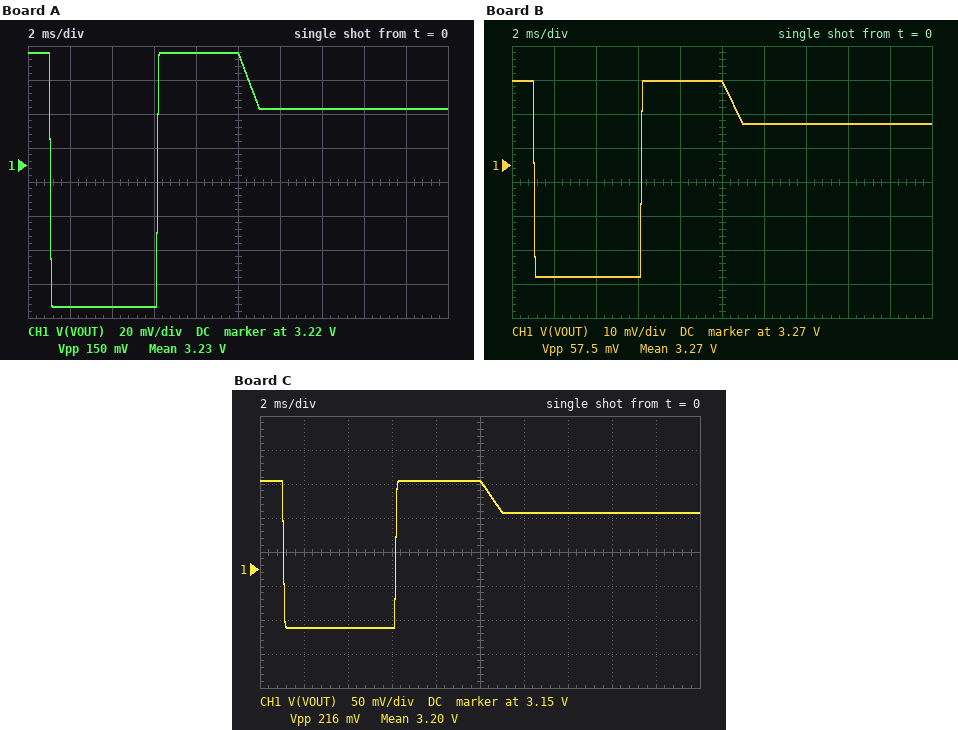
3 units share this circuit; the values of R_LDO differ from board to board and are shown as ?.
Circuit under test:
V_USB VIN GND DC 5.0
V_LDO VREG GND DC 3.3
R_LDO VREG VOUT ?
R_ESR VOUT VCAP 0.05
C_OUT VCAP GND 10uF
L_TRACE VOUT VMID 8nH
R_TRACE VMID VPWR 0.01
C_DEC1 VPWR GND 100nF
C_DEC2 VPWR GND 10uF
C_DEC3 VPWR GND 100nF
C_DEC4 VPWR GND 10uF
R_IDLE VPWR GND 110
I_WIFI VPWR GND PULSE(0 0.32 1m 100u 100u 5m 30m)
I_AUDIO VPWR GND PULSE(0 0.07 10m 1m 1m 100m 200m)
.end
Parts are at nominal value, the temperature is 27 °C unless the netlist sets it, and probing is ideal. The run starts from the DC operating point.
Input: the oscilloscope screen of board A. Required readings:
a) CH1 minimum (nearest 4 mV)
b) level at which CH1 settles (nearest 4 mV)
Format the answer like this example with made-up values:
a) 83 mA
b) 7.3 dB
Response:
a) 3.136 V
b) 3.252 V
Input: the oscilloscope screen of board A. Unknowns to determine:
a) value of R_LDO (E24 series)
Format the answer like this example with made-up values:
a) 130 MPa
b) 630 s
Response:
a) 0.47 Ω
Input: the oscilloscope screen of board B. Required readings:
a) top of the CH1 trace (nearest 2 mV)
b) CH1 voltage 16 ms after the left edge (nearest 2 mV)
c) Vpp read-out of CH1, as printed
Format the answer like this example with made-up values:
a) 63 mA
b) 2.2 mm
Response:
a) 3.294 V
b) 3.282 V
c) 57.5 mV
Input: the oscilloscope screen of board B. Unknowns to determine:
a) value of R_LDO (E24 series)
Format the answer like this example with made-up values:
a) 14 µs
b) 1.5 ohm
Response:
a) 0.18 Ω
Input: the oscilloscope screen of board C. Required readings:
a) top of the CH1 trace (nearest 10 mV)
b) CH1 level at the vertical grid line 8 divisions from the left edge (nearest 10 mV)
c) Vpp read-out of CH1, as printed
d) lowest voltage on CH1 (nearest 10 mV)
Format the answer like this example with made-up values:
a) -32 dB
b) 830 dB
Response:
a) 3.28 V
b) 3.23 V
c) 216 mV
d) 3.06 V
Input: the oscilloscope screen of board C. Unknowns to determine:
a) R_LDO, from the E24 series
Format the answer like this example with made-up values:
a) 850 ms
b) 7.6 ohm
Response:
a) 0.68 Ω
